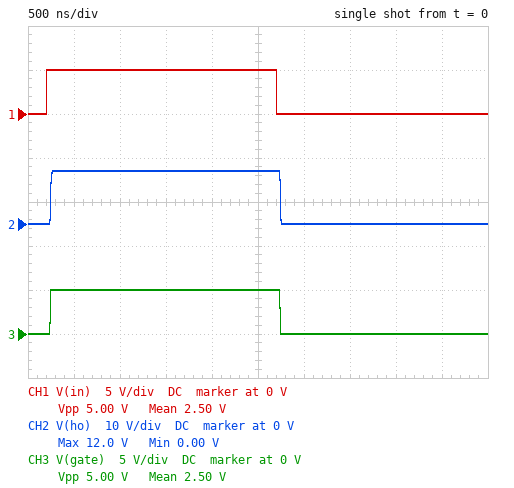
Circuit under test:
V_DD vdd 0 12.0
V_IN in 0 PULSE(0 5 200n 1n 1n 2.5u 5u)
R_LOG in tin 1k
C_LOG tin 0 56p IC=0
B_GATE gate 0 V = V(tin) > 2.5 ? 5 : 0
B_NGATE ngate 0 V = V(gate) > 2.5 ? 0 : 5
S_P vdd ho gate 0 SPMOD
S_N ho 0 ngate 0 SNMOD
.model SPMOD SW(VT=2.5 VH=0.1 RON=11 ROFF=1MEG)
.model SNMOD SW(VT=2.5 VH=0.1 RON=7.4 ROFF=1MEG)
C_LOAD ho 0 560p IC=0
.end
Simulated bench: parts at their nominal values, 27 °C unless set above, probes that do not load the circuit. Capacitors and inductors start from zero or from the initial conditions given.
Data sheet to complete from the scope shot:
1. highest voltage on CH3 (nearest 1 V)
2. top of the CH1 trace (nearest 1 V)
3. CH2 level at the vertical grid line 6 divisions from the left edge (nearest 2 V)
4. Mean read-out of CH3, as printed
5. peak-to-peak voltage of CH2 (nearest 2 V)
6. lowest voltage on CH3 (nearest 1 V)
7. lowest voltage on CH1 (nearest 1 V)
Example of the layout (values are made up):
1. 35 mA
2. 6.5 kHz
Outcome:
1. 5 V
2. 5 V
3. 0 V
4. 2.50 V
5. 12 V
6. 0 V
7. 0 V
